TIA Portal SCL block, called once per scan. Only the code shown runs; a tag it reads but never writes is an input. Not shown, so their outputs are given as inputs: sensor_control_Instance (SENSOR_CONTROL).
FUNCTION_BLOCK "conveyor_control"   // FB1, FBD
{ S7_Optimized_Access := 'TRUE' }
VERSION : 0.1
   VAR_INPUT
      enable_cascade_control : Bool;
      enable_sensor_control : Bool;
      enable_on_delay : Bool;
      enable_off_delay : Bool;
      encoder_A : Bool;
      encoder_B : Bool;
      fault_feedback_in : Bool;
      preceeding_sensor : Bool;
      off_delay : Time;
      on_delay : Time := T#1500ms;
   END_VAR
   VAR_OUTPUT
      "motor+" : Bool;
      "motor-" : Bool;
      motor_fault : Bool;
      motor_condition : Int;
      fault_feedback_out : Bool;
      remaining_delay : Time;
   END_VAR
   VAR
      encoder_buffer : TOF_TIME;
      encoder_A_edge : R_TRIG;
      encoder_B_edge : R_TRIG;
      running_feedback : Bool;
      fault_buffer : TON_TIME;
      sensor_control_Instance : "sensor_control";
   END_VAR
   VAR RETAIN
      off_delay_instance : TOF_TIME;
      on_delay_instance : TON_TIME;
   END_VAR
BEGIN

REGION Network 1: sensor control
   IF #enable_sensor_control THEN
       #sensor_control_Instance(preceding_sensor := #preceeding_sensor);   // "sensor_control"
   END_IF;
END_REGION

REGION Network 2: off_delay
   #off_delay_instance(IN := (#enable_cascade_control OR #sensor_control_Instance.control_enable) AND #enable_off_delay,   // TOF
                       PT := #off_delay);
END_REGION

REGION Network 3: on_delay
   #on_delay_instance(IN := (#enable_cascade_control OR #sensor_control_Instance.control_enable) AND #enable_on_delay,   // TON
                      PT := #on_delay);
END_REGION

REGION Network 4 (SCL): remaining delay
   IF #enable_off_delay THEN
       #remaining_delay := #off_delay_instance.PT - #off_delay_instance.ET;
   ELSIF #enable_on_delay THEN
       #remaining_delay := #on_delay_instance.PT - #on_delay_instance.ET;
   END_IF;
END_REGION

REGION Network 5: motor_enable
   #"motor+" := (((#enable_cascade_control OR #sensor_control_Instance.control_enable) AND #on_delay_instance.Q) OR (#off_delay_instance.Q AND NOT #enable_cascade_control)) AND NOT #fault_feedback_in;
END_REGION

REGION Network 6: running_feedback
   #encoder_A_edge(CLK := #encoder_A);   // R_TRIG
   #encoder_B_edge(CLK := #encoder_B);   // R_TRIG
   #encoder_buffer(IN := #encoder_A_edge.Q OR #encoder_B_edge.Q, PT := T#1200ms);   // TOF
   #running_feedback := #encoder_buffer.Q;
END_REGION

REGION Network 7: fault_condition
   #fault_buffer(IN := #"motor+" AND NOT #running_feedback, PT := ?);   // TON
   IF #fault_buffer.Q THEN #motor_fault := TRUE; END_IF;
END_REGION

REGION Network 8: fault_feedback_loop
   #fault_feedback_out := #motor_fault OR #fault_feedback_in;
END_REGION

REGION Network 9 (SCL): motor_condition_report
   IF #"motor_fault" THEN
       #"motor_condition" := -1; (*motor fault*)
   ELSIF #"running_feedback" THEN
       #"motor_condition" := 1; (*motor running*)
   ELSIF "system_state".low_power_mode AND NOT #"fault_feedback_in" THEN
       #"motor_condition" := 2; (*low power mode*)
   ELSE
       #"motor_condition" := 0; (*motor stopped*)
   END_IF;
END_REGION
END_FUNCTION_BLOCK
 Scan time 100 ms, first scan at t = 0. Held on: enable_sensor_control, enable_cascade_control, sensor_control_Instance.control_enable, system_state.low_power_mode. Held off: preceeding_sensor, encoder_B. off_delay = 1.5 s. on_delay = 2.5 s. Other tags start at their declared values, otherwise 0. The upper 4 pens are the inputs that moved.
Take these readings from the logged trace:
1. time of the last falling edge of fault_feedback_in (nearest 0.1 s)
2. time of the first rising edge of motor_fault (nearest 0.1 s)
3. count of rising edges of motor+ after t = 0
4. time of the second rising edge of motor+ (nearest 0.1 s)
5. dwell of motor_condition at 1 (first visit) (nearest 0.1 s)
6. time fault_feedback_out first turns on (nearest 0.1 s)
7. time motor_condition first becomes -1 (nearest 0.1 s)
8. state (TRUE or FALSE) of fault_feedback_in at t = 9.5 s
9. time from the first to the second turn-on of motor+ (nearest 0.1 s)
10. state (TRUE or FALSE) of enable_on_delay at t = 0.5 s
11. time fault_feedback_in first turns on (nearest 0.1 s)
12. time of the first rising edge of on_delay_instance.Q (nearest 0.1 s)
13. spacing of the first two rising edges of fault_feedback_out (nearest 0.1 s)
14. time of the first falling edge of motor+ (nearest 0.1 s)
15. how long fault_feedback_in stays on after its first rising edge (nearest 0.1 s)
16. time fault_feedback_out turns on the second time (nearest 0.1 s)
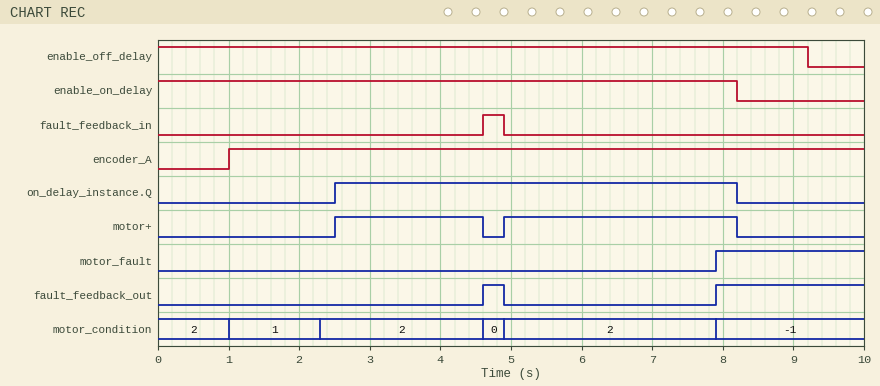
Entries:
4.9 s
7.9 s
2
4.9 s
1.3 s
4.6 s
7.9 s
FALSE
2.4 s
TRUE
4.6 s
2.5 s
3.3 s
4.6 s
0.3 s
7.9 s
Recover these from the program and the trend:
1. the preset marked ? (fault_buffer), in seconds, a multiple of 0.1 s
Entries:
3.0 s
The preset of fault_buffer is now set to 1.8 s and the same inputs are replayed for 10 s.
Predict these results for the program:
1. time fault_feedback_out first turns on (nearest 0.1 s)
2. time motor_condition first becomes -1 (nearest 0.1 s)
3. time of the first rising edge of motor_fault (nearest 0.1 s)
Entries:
4.3 s
4.3 s
4.3 s
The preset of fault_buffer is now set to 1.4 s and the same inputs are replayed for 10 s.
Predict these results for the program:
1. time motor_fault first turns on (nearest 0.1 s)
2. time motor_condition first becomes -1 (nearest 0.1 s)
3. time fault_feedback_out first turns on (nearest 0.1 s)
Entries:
3.9 s
3.9 s
3.9 s
